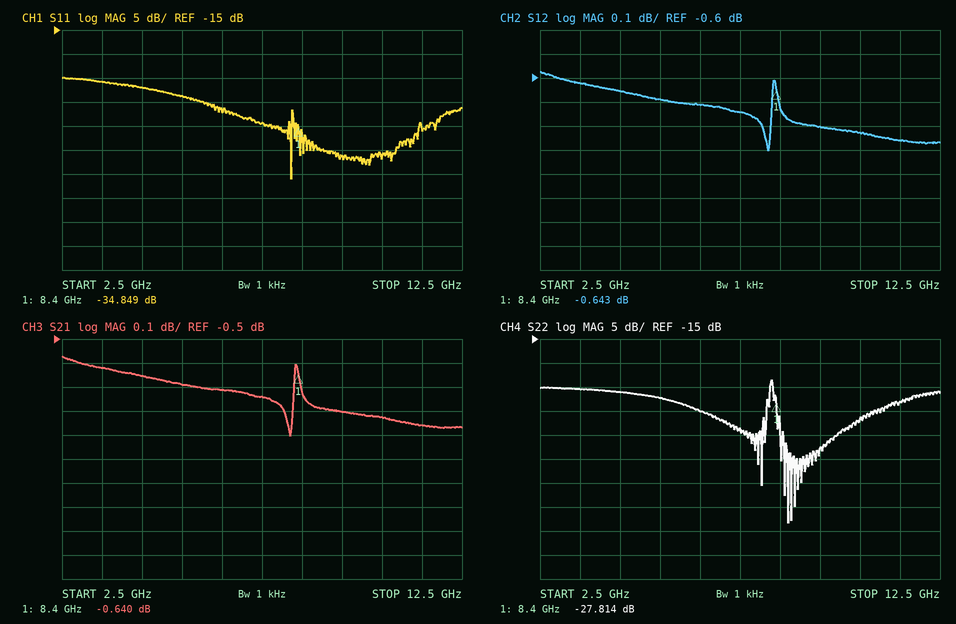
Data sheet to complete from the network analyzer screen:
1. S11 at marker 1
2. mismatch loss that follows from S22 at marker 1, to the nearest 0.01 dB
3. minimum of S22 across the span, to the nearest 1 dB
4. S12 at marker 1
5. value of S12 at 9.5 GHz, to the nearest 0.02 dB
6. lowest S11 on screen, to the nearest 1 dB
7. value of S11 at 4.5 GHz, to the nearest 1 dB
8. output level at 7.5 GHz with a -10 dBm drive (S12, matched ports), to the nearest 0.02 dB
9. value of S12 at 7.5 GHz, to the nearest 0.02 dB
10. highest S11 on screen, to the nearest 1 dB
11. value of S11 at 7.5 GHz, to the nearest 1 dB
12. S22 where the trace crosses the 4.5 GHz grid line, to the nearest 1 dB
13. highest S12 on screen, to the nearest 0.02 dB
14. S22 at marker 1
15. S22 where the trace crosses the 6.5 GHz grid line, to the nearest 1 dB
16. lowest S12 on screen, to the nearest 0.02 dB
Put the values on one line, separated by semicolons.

-34.849 dB; 0.01 dB; -53 dB; -0.643 dB; -0.80 dB; -46 dB; -27 dB; -10.74 dBm; -0.74 dB; -25 dB; -34 dB; -26 dB; -0.58 dB; -27.814 dB; -30 dB; -0.90 dB
